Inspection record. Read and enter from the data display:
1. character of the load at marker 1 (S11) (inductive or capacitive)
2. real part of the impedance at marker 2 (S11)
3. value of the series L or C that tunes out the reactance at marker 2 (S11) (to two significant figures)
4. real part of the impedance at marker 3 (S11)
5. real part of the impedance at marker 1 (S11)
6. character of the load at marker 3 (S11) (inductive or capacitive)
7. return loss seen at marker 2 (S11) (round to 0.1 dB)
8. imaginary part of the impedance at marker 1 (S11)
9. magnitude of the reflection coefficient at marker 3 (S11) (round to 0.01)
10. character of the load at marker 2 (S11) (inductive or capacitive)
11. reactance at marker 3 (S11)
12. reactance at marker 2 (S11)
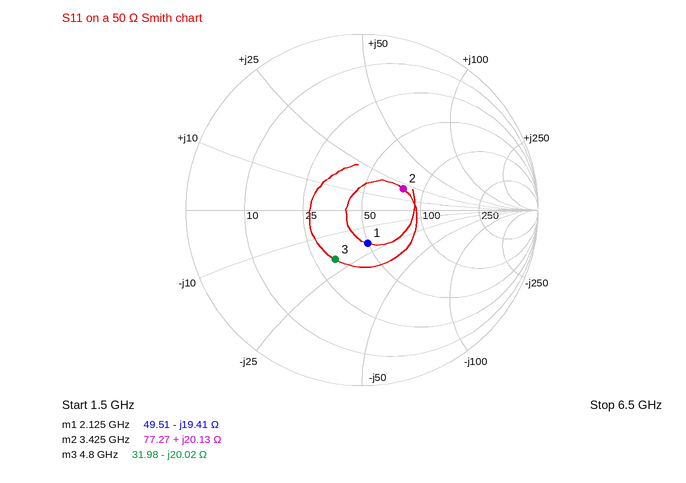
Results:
capacitive
77.27 Ω
2.3 pF
31.98 Ω
49.51 Ω
capacitive
11.6 dB
-19.41 Ω
0.32
inductive
-20.02 Ω
+20.13 Ω
